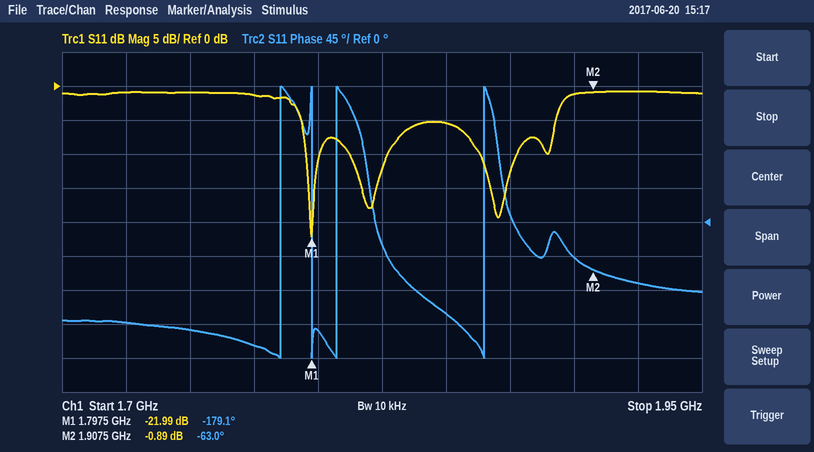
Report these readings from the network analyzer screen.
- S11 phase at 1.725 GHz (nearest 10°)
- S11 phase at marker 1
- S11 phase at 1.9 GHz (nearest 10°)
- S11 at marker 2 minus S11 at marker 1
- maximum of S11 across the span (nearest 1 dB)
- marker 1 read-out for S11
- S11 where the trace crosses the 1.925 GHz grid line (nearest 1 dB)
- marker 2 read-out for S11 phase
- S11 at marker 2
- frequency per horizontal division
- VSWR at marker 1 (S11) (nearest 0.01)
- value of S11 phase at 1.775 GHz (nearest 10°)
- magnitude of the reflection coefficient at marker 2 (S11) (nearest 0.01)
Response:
-130°
-179.1°
-50°
21.10 dB
-1 dB
-21.99 dB
-1 dB
-63.0°
-0.89 dB
25 MHz
1.17
-160°
0.90
